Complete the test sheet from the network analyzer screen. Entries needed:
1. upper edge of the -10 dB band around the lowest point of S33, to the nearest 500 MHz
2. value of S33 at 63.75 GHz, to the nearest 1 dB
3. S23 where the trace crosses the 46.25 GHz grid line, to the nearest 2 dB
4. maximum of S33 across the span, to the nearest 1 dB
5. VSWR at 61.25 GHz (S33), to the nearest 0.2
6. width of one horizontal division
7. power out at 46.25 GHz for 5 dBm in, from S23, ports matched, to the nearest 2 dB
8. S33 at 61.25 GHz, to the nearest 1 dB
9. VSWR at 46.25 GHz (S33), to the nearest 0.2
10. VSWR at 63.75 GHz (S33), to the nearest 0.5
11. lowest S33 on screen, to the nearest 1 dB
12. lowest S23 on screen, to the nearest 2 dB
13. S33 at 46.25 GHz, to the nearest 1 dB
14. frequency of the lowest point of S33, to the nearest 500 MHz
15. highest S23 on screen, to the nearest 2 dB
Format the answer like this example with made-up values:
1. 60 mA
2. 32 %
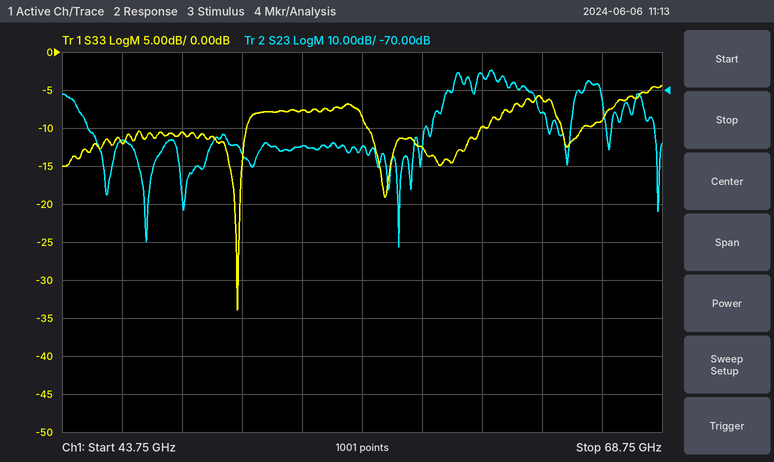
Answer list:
1. 51.5 GHz
2. -6 dB
3. -84 dB
4. -4 dB
5. 2.0
6. 2.5 GHz
7. -78 dBm
8. -10 dB
9. 1.6
10. 3.0
11. -34 dB
12. -112 dB
13. -12 dB
14. 51.0 GHz
15. -64 dB
